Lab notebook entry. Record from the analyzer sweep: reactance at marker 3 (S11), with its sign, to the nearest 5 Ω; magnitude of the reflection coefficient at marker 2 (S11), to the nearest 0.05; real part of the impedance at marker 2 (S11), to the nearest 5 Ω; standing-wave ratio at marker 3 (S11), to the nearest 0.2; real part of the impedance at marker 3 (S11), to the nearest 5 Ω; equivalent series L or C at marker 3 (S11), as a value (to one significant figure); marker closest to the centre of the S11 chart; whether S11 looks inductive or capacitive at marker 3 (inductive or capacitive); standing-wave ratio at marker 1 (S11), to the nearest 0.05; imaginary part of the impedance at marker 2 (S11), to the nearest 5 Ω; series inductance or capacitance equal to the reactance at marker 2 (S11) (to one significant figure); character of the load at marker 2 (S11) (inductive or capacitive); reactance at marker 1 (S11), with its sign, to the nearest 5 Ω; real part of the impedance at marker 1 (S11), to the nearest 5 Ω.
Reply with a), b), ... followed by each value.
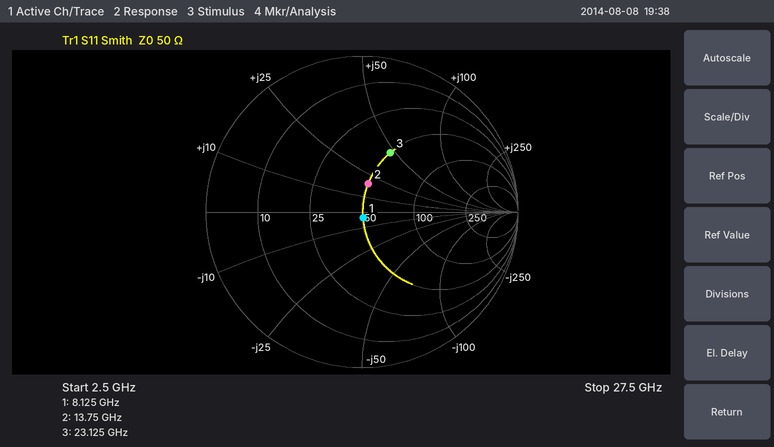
a) +45 Ω
b) 0.20
c) 50 Ω
d) 2.4
e) 50 Ω
f) 300 pH
g) marker 1
h) inductive
i) 1.10
j) +20 Ω
k) 200 pH
l) inductive
m) -5 Ω
n) 50 Ω
